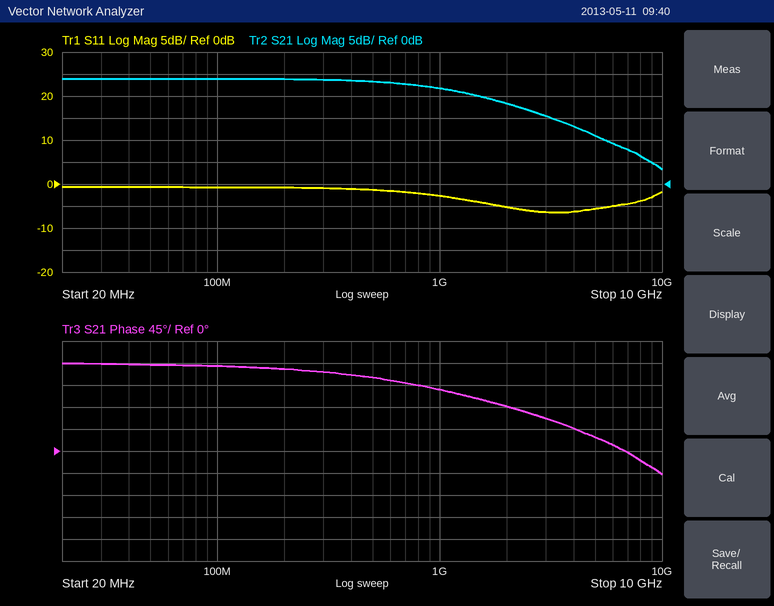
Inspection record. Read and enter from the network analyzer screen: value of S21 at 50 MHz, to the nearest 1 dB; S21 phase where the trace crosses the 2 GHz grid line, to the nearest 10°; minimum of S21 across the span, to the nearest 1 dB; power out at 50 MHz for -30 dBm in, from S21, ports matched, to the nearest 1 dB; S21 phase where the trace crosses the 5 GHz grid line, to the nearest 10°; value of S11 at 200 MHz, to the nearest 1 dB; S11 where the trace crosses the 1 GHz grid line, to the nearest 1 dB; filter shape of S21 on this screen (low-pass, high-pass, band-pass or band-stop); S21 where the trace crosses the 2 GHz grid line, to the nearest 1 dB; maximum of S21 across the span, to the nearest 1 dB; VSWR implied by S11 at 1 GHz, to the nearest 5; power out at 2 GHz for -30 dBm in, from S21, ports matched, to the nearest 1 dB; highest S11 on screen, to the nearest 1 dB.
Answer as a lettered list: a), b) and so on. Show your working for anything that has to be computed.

a) 24 dB
b) 90°
c) 3 dB
d) -30 dBm + (24 dB) = -6 dBm
e) 30°
f) -1 dB
g) -3 dB
h) low-pass
i) 18 dB
j) 24 dB
k) |Γ| = 10^(-3/20) = 0.7079; VSWR = (1 + 0.7079)/(1 − 0.7079) ≈ 5.85, so 5 to the nearest 5
l) -30 dBm + (18 dB) = -12 dBm
m) -1 dB
